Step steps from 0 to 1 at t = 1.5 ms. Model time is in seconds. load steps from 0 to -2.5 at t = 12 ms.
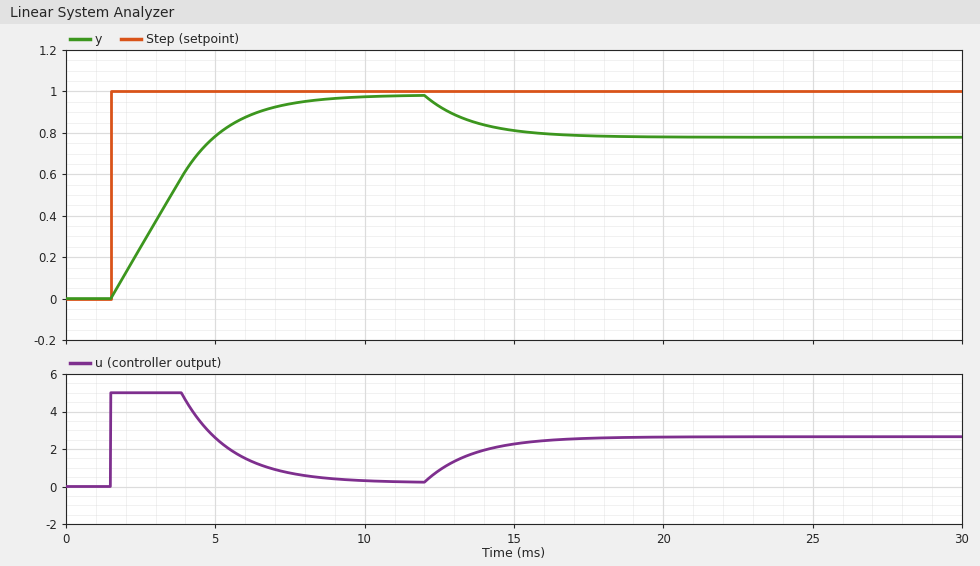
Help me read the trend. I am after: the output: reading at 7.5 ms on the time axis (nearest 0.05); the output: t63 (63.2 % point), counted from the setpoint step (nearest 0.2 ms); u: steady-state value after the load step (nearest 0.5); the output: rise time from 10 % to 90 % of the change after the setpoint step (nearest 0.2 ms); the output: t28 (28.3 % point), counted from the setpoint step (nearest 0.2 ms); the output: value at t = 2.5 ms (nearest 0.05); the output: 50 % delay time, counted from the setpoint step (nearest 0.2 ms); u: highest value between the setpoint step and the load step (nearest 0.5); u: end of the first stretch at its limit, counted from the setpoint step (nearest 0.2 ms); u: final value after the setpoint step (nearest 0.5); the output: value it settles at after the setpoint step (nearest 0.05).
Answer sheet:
0.95
2.6 ms
2.5
4.2 ms
1.2 ms
0.25
2.0 ms
5.0
2.4 ms
0.0
1.00
